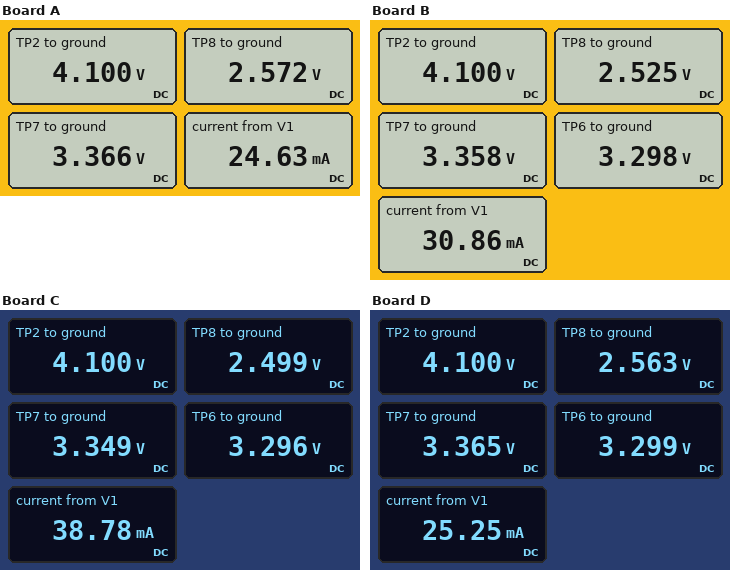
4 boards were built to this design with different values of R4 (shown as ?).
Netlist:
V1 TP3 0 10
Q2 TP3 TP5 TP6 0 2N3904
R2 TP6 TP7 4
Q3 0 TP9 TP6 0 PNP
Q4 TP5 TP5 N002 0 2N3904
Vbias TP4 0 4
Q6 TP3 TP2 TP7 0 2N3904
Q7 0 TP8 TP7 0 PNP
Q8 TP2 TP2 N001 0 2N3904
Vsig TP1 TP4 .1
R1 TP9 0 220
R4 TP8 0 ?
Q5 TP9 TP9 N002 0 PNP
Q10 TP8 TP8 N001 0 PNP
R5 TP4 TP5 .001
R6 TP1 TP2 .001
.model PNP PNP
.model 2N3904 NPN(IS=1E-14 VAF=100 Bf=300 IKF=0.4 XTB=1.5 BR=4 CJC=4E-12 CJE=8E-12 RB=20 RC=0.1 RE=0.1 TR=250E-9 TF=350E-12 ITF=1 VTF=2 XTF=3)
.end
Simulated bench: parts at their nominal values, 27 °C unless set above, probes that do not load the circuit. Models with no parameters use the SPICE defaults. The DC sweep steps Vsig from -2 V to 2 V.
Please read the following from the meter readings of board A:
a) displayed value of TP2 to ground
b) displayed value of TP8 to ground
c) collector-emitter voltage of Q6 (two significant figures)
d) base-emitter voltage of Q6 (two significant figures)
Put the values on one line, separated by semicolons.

4.100 V; 2.572 V; 6.6 V; 730 mV
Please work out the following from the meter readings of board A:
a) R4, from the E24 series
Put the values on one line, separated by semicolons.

390 Ω
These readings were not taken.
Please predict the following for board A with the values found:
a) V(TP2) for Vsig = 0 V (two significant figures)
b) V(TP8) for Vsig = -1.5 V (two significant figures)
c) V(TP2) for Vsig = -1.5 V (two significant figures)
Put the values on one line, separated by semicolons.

4.0 V; 1.1 V; 2.5 V
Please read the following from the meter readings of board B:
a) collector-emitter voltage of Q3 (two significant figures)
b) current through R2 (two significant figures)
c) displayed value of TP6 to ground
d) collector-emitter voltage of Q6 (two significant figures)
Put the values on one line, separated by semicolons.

-3.3 V; 15 mA; 3.298 V; 6.6 V
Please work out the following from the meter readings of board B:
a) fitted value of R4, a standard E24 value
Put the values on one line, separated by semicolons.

160 Ω
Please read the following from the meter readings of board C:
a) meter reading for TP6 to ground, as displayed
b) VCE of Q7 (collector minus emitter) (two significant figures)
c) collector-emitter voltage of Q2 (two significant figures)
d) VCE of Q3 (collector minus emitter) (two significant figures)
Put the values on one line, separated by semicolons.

3.296 V; -3.3 V; 6.7 V; -3.3 V
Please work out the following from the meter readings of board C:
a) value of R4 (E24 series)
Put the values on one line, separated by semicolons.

100 Ω
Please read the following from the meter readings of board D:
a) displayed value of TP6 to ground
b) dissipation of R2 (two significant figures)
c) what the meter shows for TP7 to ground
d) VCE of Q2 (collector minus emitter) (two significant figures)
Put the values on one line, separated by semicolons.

3.299 V; 1.1 mW; 3.365 V; 6.7 V
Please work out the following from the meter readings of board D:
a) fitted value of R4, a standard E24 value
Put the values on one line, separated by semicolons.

330 Ω
